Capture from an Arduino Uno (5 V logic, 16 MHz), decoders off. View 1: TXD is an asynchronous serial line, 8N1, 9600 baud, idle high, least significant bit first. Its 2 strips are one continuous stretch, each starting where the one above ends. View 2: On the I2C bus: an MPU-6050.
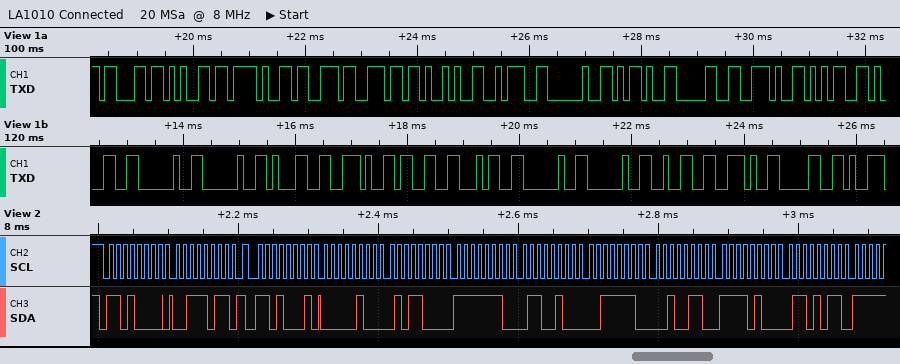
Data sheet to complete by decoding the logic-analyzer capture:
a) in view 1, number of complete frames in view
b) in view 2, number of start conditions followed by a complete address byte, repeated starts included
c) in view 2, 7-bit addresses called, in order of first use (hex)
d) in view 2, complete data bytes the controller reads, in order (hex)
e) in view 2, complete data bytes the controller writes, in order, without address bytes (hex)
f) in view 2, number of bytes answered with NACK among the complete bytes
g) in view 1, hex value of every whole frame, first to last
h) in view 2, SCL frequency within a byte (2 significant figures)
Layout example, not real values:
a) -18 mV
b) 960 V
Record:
a) 24
b) 2
c) 0x68
d) 04 58 FE 64 3E 26 F4 6B
e) 3B
f) 0
g) 63 65 2F 73 6E 29 3A 20 2D 30 2E 35 31 20 20 31 2E 33 34 20 20 32 2E 30
h) 100 kHz
